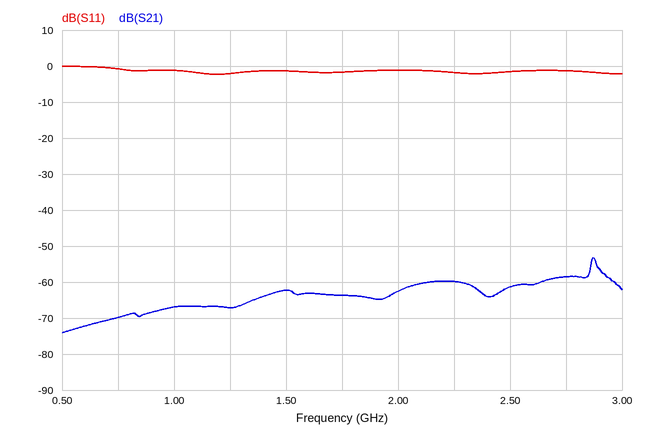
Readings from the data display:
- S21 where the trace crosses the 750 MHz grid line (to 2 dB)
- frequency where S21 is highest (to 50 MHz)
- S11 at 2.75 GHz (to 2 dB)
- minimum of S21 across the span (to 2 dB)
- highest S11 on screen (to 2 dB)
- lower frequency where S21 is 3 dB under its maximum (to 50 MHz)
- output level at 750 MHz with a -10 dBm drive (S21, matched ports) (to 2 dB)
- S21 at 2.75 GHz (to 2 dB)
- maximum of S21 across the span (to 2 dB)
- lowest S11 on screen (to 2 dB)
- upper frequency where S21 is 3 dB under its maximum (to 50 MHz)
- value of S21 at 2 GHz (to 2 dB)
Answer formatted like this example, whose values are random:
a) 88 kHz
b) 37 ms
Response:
a) -70 dB
b) 2.85 GHz
c) -2 dB
d) -74 dB
e) 0 dB
f) 2.85 GHz
g) -80 dBm
h) -58 dB
i) -54 dB
j) -2 dB
k) 2.90 GHz
l) -62 dB
